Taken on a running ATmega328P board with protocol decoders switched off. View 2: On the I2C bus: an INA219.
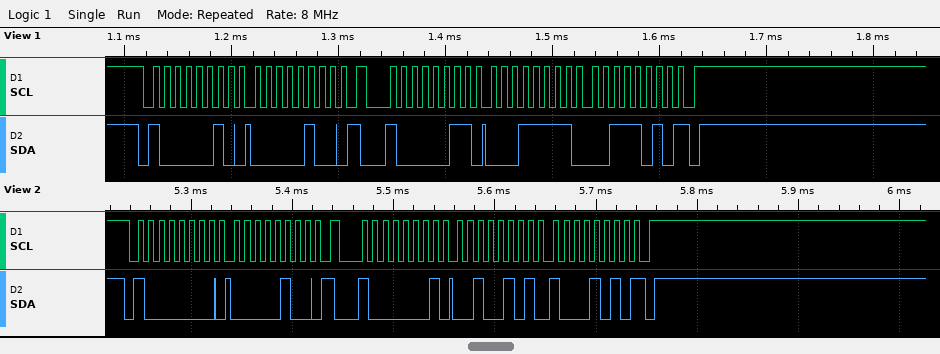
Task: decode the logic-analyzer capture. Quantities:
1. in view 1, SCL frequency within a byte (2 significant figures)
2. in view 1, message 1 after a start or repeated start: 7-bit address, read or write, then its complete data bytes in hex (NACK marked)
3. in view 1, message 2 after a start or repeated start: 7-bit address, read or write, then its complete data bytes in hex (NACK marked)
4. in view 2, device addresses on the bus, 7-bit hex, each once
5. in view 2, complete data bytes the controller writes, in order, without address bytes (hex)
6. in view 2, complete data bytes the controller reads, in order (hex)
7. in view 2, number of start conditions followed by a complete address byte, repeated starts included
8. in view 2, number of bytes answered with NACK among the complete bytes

100 kHz
0x41 write: 04
0x41 read: 1F 3A NACK
0x40
04
25 8A
2
1
